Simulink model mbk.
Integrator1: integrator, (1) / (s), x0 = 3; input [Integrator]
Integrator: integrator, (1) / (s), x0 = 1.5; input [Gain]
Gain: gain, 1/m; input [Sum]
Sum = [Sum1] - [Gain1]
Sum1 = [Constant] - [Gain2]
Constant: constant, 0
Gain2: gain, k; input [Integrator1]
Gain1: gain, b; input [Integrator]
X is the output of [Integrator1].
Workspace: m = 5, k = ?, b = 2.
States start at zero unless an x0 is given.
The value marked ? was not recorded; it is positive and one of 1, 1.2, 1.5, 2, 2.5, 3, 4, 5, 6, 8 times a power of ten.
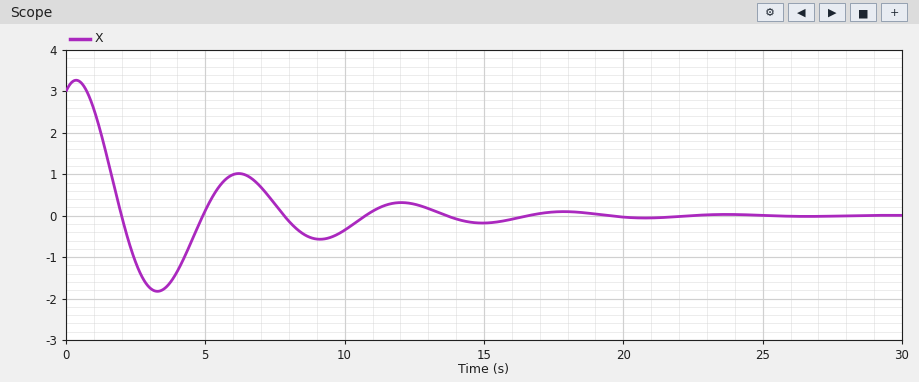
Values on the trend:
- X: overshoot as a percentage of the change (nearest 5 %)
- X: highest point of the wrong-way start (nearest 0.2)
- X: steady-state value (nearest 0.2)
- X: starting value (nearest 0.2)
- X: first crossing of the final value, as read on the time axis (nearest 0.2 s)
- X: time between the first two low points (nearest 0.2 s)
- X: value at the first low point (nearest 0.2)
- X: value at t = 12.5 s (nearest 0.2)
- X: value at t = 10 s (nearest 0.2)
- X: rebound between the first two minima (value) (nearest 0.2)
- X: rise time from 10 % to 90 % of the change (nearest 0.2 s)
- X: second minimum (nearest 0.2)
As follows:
60 %
3.2
0.0
3.0
2.0 s
5.8 s
-1.8
0.2
-0.4
1.0
1.0 s
-0.6
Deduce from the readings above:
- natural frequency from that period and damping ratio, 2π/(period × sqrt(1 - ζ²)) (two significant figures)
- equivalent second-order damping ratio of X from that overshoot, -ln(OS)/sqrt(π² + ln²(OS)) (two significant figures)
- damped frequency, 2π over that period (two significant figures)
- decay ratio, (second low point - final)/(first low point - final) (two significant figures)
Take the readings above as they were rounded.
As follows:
1.1 rad/s
0.16
1.1 rad/s
0.33
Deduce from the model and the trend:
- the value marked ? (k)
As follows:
6
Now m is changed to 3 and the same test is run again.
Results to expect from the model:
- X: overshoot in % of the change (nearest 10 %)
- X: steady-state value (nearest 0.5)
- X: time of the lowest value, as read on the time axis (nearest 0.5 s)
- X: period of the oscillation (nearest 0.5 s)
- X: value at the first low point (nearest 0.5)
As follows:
50 %
0.0
2.5 s
4.5 s
-1.5
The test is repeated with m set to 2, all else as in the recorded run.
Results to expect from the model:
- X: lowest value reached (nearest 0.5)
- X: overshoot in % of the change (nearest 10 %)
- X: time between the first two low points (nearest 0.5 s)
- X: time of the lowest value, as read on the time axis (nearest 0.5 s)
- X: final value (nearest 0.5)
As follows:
-1.0
40 %
4.0 s
2.0 s
0.0
